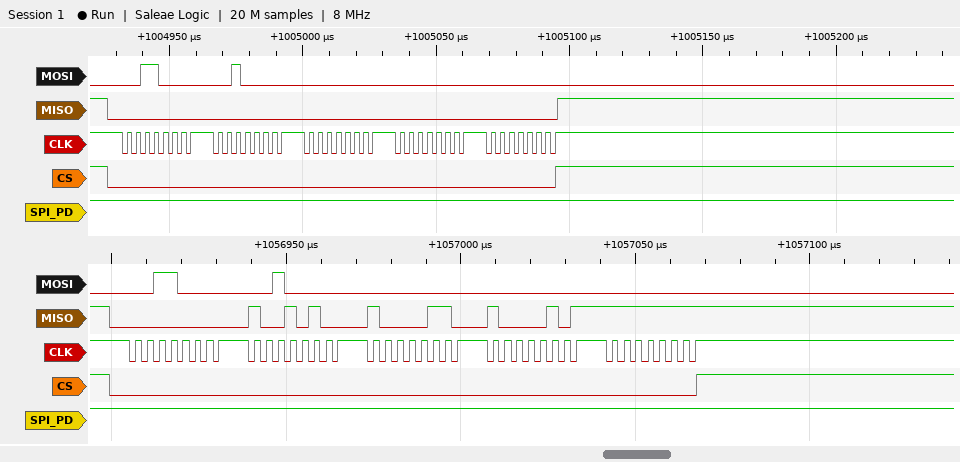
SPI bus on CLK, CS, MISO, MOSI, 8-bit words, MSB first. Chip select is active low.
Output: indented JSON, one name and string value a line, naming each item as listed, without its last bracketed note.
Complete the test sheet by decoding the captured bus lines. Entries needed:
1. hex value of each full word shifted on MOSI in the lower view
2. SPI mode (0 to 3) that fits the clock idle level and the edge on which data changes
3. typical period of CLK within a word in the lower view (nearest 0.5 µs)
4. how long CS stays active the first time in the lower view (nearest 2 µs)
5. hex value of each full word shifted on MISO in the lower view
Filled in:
{
  "hex value of each full word shifted on MOSI in the lower view": "30, 20, 00, 00, 00",
  "SPI mode (0 to 3) that fits the clock idle level and the edge on which data changes": "3",
  "typical period of CLK within a word in the lower view": "3.5 µs",
  "how long CS stays active the first time in the lower view": "168 µs",
  "hex value of each full word shifted on MISO in the lower view": "00, 94, 86, 85, FF"
}
